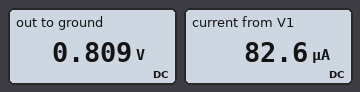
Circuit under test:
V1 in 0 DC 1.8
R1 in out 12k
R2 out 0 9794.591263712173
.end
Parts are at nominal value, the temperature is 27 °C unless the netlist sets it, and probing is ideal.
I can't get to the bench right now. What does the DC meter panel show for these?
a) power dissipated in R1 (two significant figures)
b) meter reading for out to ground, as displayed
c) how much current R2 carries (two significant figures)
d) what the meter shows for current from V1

82 µW
0.809 V
83 µA
82.6 µA
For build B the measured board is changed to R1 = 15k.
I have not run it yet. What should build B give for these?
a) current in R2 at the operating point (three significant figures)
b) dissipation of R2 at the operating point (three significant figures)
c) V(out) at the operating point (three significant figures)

72.6 µA
51.6 µW
711 mV
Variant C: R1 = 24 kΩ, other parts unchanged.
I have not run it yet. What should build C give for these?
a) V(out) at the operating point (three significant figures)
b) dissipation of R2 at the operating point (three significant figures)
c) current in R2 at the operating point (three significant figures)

522 mV
27.8 µW
53.3 µA
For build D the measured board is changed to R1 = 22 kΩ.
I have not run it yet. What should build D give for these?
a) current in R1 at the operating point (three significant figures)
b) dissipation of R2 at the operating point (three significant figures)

56.6 µA
31.4 µW
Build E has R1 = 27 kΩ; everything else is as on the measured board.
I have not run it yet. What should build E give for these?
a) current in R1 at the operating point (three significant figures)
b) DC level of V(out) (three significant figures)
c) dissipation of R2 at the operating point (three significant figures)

48.9 µA
479 mV
23.4 µW
